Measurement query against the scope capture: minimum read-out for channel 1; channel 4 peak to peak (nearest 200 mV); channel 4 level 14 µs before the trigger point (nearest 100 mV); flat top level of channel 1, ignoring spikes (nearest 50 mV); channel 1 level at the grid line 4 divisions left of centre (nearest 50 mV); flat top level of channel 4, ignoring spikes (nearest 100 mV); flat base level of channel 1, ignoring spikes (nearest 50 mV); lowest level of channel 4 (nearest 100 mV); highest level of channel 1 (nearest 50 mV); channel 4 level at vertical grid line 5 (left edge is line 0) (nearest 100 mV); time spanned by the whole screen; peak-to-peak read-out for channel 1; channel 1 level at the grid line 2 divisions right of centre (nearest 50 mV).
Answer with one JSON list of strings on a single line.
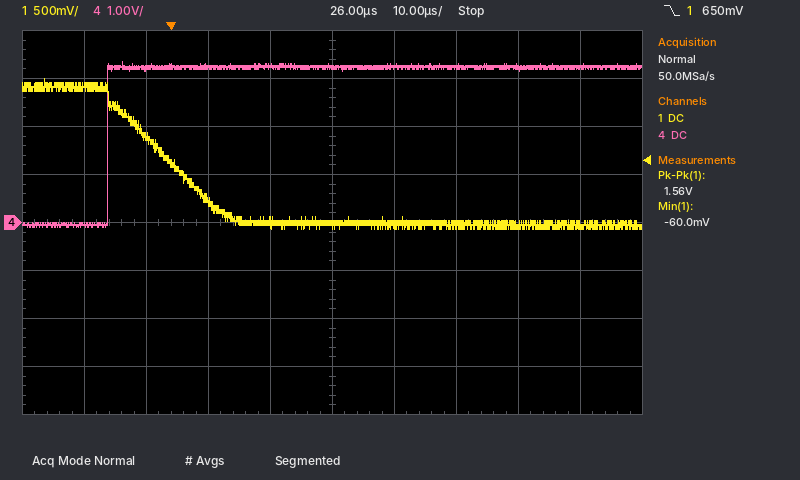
["-60.0 mV", "3.4 V", "0.0 V", "1.40 V", "1.40 V", "3.2 V", "0 mV", "-100 mV", "1.50 V", "3.2 V", "100 µs", "1.56 V", "0 mV"]
